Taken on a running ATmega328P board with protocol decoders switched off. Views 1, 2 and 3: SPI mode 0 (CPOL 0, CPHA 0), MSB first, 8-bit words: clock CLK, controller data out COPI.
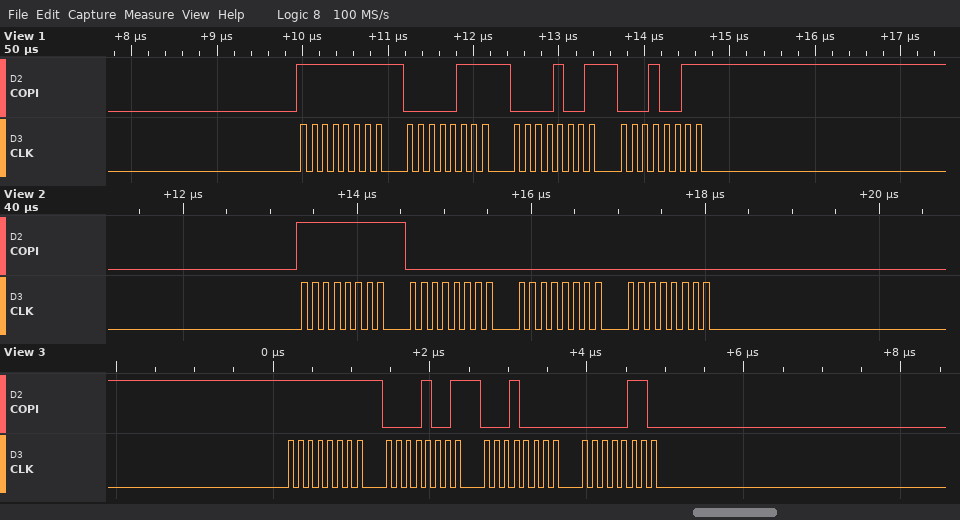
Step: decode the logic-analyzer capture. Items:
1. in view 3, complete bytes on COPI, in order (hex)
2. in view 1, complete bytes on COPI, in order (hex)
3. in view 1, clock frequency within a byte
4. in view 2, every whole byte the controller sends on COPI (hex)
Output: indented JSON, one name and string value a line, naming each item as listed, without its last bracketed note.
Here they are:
{
  "in view 3, complete bytes on COPI, in order": "FF 09 10 06",
  "in view 1, complete bytes on COPI, in order": "FF 07 09 13",
  "in view 1, clock frequency within a byte": "8 MHz",
  "in view 2, every whole byte the controller sends on COPI": "FF 00 00 00"
}
